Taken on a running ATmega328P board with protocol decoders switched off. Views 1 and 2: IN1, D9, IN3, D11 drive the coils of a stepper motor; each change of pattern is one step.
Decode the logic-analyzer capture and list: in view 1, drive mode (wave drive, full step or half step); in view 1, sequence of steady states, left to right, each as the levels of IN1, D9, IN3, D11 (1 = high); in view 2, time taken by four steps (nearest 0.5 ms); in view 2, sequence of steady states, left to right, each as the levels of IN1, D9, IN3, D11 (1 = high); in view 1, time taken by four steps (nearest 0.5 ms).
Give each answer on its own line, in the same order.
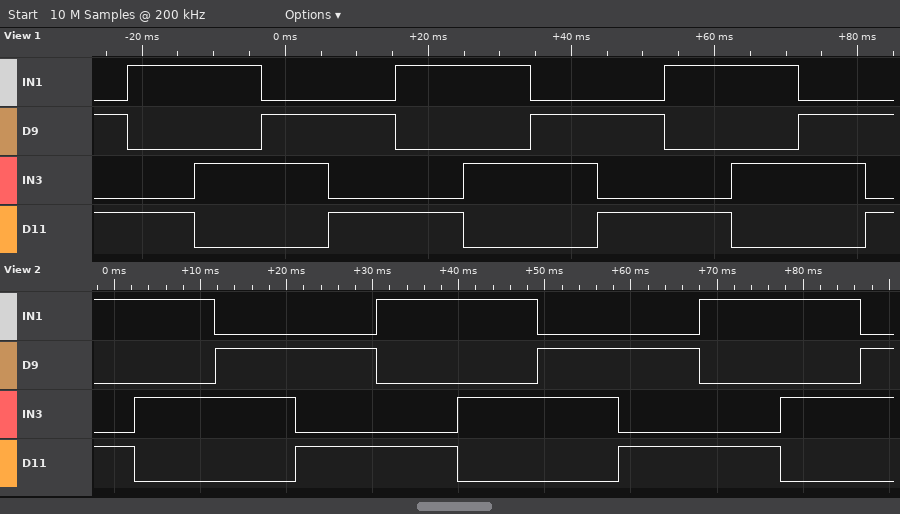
full step
0101 1001 1010 0110 0101 1001 1010 0110 0101 1001 1010 0110 0101
37.5 ms
1001 1010 0110 0101 1001 1010 0110 0101 1001 1010 0110
37.5 ms
